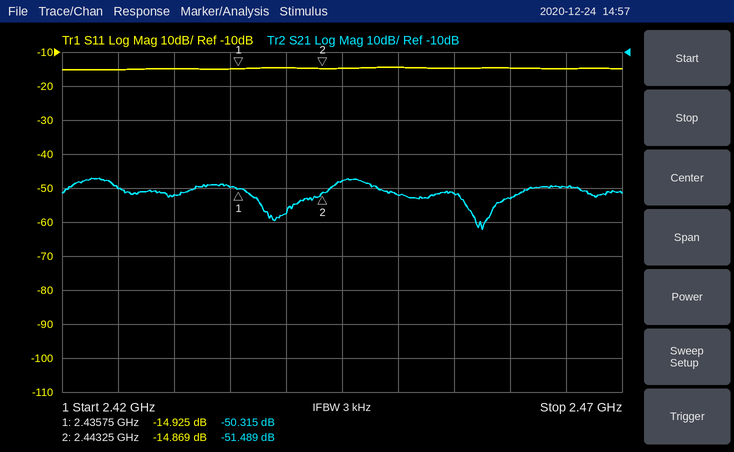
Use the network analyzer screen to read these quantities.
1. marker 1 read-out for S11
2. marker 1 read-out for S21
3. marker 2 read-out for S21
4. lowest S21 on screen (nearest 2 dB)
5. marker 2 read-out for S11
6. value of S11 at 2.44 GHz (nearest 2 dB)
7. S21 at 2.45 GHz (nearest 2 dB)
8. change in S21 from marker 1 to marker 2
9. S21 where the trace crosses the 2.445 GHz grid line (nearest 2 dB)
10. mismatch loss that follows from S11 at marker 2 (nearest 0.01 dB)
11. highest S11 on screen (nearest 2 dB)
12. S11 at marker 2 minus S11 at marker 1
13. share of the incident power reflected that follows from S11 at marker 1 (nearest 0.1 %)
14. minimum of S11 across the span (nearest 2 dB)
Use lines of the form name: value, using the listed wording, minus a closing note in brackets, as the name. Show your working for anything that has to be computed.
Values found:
marker 1 read-out for S11: -14.925 dB
marker 1 read-out for S21: -50.315 dB
marker 2 read-out for S21: -51.489 dB
lowest S21 on screen: -62 dB
marker 2 read-out for S11: -14.869 dB
value of S11 at 2.44 GHz: -14 dB
S21 at 2.45 GHz: -52 dB
change in S21 from marker 1 to marker 2: -51.489 − (-50.315) = -1.174 dB
S21 where the trace crosses the 2.445 GHz grid line: -48 dB
mismatch loss that follows from S11 at marker 2: −10 log10(1 − 10^(-14.869/10)) ≈ 0.14 dB
highest S11 on screen: -14 dB
S11 at marker 2 minus S11 at marker 1: -14.869 − (-14.925) = 0.056 dB
share of the incident power reflected that follows from S11 at marker 1: 10^(-14.925/10) ≈ 3.2 %
minimum of S11 across the span: -16 dB
